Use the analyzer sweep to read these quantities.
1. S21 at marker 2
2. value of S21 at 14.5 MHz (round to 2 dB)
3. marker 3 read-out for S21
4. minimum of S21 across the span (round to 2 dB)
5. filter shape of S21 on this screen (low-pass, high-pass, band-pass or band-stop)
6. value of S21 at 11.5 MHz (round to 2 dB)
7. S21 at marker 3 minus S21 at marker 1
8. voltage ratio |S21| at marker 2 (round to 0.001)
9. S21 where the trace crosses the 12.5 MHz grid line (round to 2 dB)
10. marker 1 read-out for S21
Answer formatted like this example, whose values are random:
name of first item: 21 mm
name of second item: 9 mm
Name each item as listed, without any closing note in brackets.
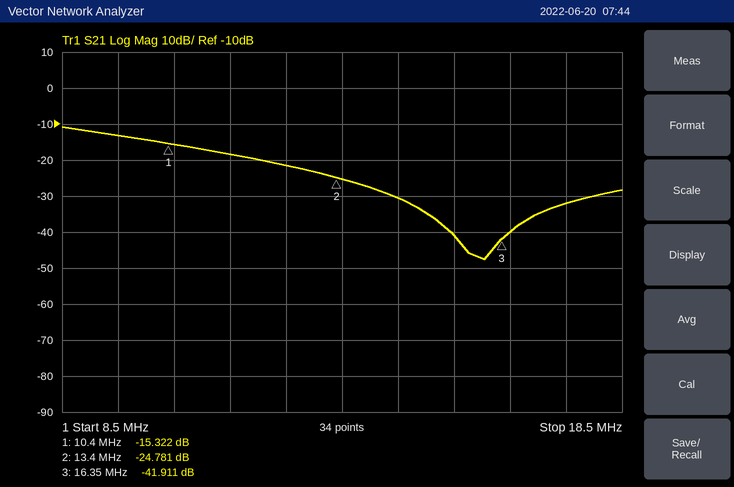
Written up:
S21 at marker 2: -24.781 dB
value of S21 at 14.5 MHz: -30 dB
marker 3 read-out for S21: -41.911 dB
minimum of S21 across the span: -48 dB
filter shape of S21 on this screen: low-pass
value of S21 at 11.5 MHz: -18 dB
S21 at marker 3 minus S21 at marker 1: -26.589 dB
voltage ratio |S21| at marker 2: 0.058
S21 where the trace crosses the 12.5 MHz grid line: -22 dB
marker 1 read-out for S21: -15.322 dB
